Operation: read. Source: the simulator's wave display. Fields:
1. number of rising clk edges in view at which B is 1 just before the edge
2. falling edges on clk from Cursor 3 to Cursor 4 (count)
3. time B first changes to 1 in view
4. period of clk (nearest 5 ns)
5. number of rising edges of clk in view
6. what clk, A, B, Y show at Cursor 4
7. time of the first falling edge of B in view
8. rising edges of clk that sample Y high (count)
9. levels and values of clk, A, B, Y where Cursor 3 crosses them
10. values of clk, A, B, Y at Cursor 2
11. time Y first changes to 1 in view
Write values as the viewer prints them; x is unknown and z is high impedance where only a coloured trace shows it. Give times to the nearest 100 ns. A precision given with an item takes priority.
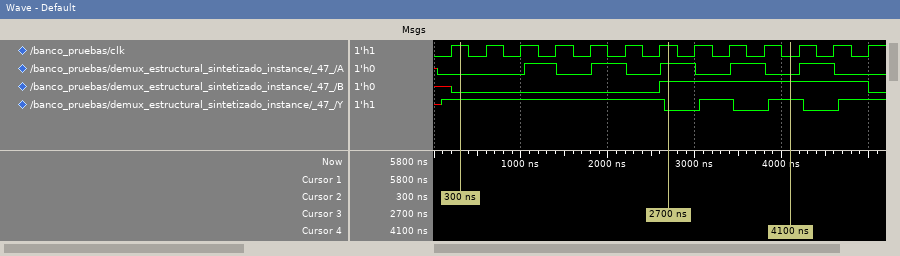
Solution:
6
4
2600 ns
400 ns
13
clk=0, A=0, B=1, Y=1
5000 ns
10
clk=1, A=1, B=1, Y=0
clk=1, A=0, B=0, Y=1
100 ns
